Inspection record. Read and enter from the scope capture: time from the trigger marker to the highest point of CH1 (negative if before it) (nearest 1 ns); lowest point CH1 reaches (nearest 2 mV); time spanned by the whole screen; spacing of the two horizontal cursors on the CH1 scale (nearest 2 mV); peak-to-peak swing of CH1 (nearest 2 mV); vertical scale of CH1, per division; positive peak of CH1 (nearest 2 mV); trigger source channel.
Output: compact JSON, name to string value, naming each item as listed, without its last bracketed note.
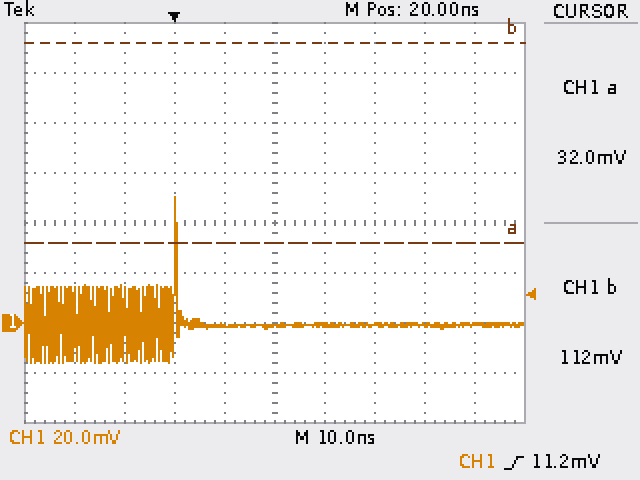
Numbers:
{"time from the trigger marker to the highest point of CH1 (negative if before it)": "0 ns", "lowest point CH1 reaches": "-16 mV", "time spanned by the whole screen": "100 ns", "spacing of the two horizontal cursors on the CH1 scale": "80 mV", "peak-to-peak swing of CH1": "66 mV", "vertical scale of CH1, per division": "20 mV", "positive peak of CH1": "50 mV", "trigger source channel": "CH1"}
